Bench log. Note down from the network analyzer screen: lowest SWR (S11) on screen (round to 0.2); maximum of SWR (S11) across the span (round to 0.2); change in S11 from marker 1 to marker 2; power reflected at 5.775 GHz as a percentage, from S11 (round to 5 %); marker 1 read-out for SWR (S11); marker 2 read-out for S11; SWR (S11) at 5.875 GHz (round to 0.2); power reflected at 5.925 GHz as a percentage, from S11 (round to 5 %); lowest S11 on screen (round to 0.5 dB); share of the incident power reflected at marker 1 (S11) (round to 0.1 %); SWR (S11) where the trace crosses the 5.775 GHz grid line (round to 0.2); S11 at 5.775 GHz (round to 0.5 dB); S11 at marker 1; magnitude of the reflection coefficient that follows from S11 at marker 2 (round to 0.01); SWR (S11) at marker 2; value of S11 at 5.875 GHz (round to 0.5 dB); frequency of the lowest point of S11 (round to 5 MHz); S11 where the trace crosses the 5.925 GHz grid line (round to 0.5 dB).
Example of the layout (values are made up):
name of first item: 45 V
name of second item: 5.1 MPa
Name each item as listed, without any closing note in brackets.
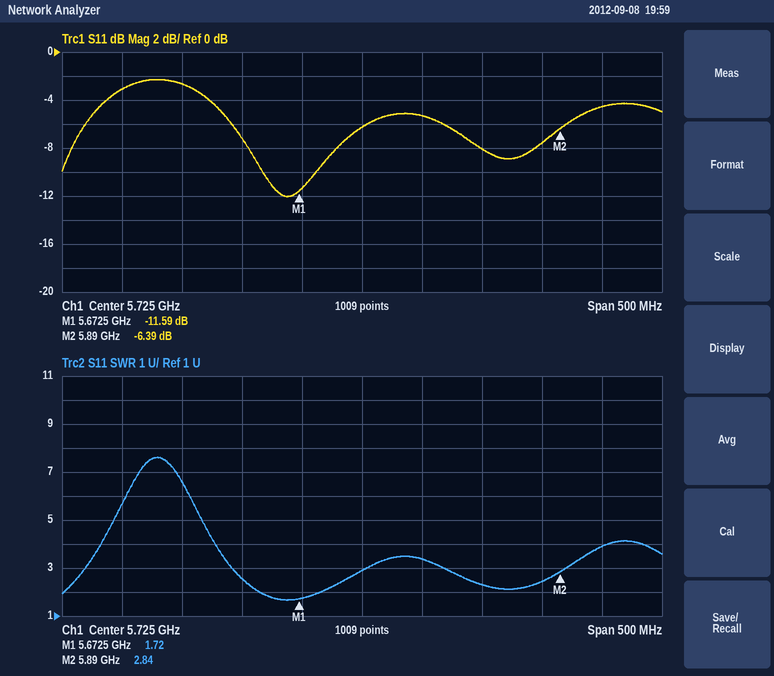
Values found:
lowest SWR (S11) on screen: 1.6
maximum of SWR (S11) across the span: 7.6
change in S11 from marker 1 to marker 2: 5.20 dB
power reflected at 5.775 GHz as a percentage, from S11: 30 %
marker 1 read-out for SWR: 1.72
marker 2 read-out for S11: -6.39 dB
SWR (S11) at 5.875 GHz: 2.4
power reflected at 5.925 GHz as a percentage, from S11: 35 %
lowest S11 on screen: -12.0 dB
share of the incident power reflected at marker 1 (S11): 6.9 %
SWR (S11) where the trace crosses the 5.775 GHz grid line: 3.4
S11 at 5.775 GHz: -5.5 dB
S11 at marker 1: -11.59 dB
magnitude of the reflection coefficient that follows from S11 at marker 2: 0.48
SWR (S11) at marker 2: 2.84
value of S11 at 5.875 GHz: -7.5 dB
frequency of the lowest point of S11: 5.660 GHz
S11 where the trace crosses the 5.925 GHz grid line: -4.5 dB
